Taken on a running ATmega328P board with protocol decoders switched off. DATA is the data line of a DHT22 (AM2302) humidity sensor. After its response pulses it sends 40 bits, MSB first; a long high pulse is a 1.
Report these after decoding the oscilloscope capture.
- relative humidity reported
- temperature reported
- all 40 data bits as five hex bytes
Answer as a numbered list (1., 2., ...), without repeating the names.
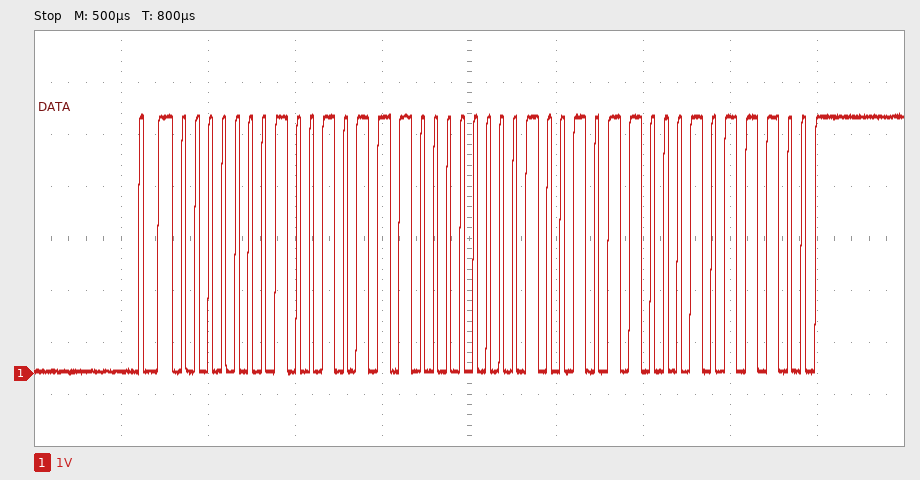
1. 30.2 %
2. 30.0 °C
3. 01 2E 01 2C 5C
